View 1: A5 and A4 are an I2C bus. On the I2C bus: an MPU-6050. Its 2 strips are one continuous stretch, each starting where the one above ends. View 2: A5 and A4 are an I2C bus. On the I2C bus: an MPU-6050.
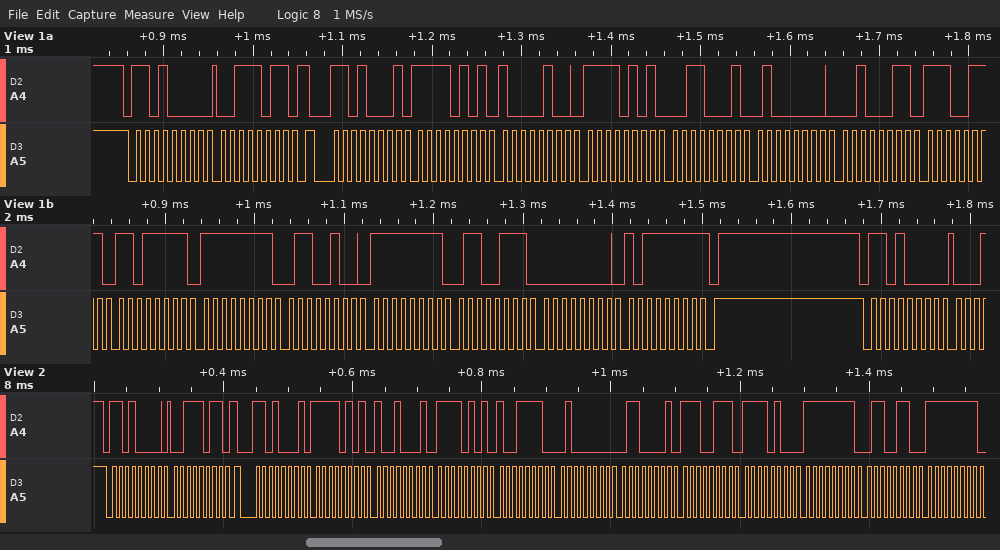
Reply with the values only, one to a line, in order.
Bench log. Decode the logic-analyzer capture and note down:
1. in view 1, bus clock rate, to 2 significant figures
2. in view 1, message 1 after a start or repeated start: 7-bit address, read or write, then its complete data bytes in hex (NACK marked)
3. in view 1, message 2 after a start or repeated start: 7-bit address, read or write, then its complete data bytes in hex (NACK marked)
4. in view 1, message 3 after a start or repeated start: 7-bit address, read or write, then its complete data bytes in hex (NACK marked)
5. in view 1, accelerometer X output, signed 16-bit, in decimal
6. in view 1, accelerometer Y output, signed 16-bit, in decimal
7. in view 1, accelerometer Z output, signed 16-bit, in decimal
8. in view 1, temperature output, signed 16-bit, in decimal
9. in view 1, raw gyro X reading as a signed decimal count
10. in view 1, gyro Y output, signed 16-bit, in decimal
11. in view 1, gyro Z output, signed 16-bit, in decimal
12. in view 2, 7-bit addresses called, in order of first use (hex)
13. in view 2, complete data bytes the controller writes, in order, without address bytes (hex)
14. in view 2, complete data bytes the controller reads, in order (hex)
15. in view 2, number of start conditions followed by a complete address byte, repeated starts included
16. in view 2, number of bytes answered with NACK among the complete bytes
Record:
100 kHz
0x68 write: 3B
0x68 read: F5 84 F5 31 40 23 E7 DF FF 64 FF 67 00 BF NACK
0x68 write
-2684
-2767
16419
-6177
-156
-153
191
0x68
3B
F5 91 F5 9E 40 61 E7 F4 FF 66 FF
2
0
